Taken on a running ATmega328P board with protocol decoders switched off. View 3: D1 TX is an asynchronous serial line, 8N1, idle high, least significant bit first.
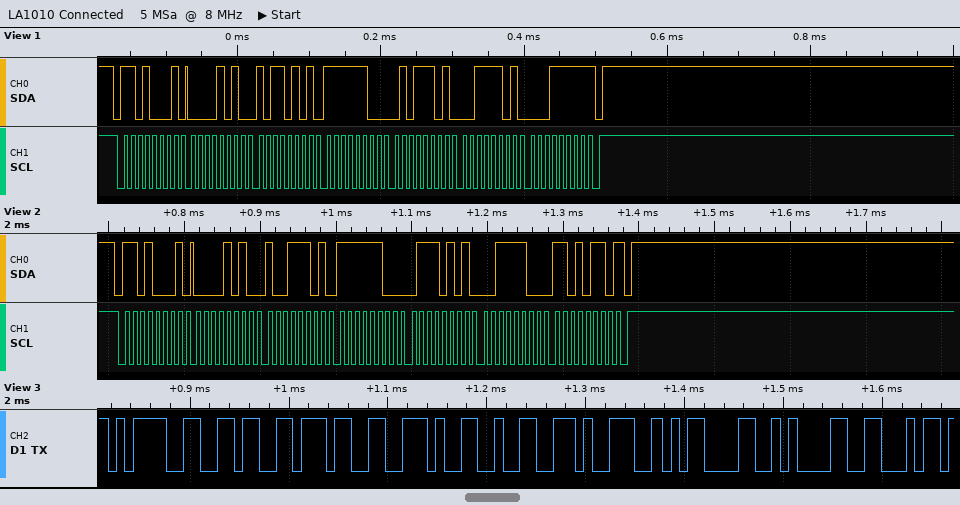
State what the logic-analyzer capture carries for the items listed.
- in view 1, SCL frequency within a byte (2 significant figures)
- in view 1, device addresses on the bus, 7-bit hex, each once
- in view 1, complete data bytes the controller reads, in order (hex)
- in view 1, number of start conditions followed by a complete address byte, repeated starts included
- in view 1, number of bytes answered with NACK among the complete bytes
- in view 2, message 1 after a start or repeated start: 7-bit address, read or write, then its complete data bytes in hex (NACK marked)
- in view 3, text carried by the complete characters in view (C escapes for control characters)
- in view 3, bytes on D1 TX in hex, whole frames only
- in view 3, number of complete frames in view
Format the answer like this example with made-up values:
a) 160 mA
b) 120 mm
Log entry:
a) 100 kHz
b) 0x68
c) 0A B5 FC 5D 3D 1F
d) 1
e) 1
f) 0x68 read: 0A 9D FC 75 3C D6 NACK
g) "=67.29\r\nF"
h) 3D 36 37 2E 32 39 0D 0A 46
i) 9
